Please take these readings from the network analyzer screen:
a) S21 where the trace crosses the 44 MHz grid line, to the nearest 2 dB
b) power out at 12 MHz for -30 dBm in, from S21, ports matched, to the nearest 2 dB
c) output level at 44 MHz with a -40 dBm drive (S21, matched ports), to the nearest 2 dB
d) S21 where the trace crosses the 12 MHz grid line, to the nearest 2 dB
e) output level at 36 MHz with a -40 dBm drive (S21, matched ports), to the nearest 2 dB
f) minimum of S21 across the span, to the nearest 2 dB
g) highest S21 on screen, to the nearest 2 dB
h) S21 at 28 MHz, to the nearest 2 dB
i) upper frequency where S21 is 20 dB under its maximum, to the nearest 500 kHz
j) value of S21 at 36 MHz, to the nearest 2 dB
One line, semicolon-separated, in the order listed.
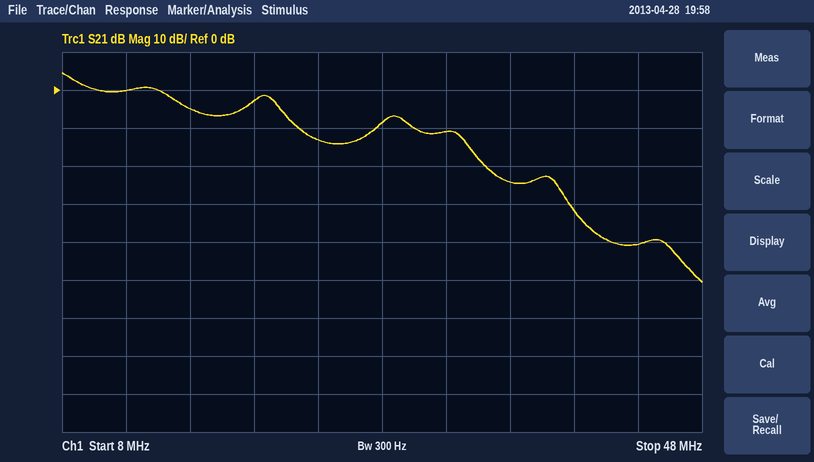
-40 dB; -30 dBm; -80 dBm; 0 dB; -64 dBm; -50 dB; 4 dB; -8 dB; 33.5 MHz; -24 dB
